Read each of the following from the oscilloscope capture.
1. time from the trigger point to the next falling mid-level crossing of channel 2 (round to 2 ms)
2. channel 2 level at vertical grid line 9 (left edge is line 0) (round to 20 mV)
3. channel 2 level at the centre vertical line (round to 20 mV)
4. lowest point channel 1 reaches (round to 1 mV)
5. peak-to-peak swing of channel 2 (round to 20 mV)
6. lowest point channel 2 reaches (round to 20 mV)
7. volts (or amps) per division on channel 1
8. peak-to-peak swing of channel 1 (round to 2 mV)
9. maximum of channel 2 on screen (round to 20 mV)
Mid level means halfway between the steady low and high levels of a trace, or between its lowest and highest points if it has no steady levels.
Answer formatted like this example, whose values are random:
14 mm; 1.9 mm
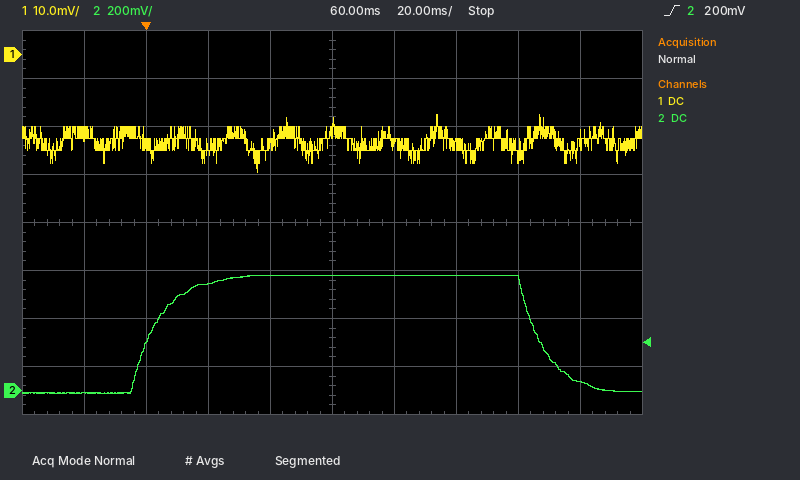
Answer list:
126 ms; 40 mV; 480 mV; -25 mV; 500 mV; -20 mV; 10 mV; 12 mV; 480 mV
